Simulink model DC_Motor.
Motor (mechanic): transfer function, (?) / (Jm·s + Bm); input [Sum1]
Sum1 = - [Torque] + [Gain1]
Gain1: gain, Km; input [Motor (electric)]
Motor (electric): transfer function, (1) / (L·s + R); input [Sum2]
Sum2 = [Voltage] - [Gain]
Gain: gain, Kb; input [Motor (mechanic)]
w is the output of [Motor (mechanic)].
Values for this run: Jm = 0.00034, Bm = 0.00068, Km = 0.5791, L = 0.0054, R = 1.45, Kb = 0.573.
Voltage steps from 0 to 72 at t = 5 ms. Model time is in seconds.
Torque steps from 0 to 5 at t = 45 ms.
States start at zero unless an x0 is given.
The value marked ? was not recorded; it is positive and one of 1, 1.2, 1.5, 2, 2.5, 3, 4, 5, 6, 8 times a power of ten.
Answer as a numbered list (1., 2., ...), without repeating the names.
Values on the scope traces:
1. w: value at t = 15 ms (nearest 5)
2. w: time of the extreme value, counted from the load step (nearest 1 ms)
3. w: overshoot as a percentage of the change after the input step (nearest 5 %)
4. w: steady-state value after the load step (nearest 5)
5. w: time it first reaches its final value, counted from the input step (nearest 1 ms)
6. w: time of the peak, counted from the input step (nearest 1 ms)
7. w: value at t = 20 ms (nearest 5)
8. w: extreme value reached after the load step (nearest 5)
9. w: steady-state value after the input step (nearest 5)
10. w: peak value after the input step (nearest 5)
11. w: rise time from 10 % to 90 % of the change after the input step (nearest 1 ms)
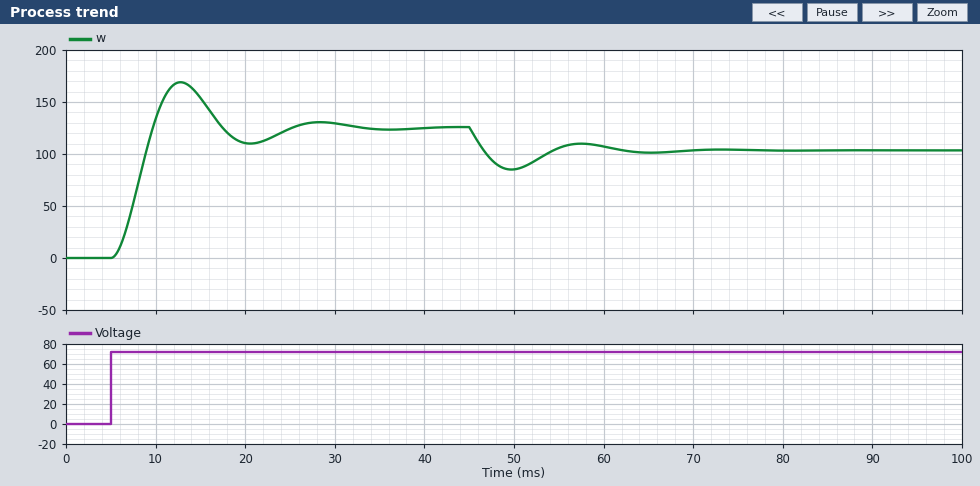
1. 155
2. 5 ms
3. 35 %
4. 105
5. 5 ms
6. 8 ms
7. 110
8. 85
9. 125
10. 170
11. 3 ms
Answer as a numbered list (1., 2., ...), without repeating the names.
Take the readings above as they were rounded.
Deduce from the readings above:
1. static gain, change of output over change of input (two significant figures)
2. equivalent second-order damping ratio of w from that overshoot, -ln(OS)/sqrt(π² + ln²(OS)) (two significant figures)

1. 1.7
2. 0.32
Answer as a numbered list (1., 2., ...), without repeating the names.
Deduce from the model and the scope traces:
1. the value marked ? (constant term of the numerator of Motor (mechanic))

1. 1
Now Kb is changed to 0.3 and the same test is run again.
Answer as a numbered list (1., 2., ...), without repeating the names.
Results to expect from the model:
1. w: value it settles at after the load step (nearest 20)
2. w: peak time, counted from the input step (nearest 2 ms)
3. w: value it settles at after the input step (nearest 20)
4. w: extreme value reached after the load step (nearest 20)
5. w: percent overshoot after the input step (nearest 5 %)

1. 200
2. 12 ms
3. 240
4. 180
5. 20 %
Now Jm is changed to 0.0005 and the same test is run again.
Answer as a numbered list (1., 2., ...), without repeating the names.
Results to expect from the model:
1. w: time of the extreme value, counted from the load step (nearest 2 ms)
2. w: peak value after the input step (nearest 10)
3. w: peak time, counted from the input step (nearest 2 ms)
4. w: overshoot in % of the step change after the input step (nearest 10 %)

1. 6 ms
2. 160
3. 10 ms
4. 30 %
